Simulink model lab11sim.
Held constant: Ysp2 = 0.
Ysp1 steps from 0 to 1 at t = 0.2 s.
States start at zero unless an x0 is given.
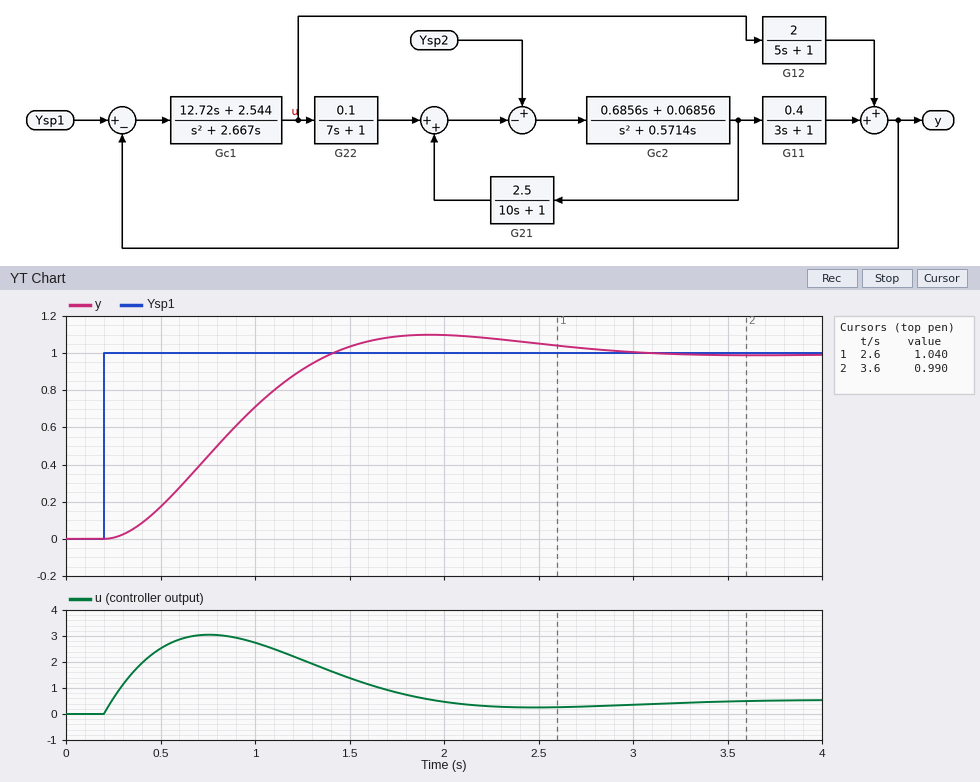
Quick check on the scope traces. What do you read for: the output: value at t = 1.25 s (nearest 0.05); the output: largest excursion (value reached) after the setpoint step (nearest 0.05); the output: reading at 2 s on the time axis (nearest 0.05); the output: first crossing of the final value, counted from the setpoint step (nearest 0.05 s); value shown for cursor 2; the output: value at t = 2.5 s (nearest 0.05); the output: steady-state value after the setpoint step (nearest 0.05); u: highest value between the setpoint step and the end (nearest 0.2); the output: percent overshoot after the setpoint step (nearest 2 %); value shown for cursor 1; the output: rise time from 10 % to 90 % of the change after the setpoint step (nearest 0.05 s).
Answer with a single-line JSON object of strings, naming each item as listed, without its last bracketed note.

{"the output: value at t = 1.25 s": "0.90", "the output: largest excursion (value reached) after the setpoint step": "1.10", "the output: reading at 2 s on the time axis": "1.10", "the output: first crossing of the final value, counted from the setpoint step": "1.20 s", "value shown for cursor 2": "0.990", "the output: value at t = 2.5 s": "1.05", "the output: steady-state value after the setpoint step": "1.00", "u: highest value between the setpoint step and the end": "3.0", "the output: percent overshoot after the setpoint step": "10 %", "value shown for cursor 1": "1.040", "the output: rise time from 10 % to 90 % of the change after the setpoint step": "0.80 s"}
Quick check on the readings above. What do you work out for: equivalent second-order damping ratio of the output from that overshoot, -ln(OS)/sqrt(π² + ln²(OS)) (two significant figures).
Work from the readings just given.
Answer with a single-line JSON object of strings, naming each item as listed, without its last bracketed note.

{"equivalent second-order damping ratio of the output from that overshoot, -ln(OS)/sqrt(π² + ln²(OS))": "0.59"}
